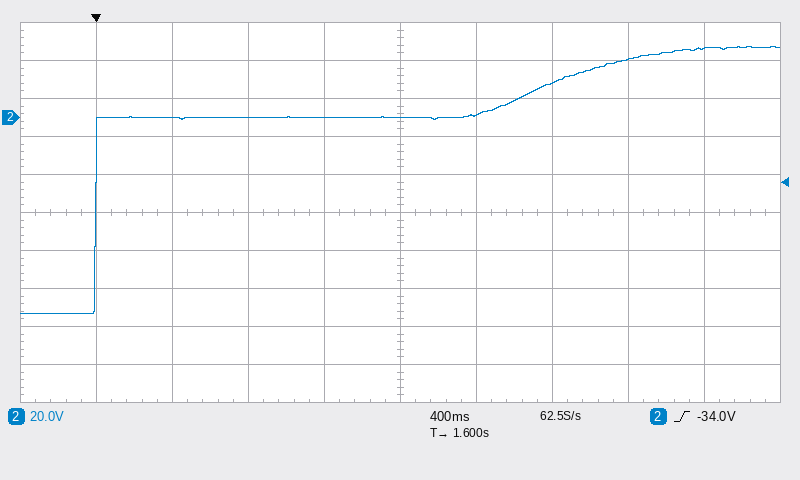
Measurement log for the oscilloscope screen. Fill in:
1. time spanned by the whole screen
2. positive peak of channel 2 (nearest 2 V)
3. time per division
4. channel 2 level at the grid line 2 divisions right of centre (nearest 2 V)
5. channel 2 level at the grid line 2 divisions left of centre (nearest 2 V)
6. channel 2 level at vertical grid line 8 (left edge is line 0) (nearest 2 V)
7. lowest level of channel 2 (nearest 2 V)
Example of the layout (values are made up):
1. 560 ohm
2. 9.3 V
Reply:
1. 4 s
2. 38 V
3. 400 ms
4. 18 V
5. 0 V
6. 30 V
7. -104 V
